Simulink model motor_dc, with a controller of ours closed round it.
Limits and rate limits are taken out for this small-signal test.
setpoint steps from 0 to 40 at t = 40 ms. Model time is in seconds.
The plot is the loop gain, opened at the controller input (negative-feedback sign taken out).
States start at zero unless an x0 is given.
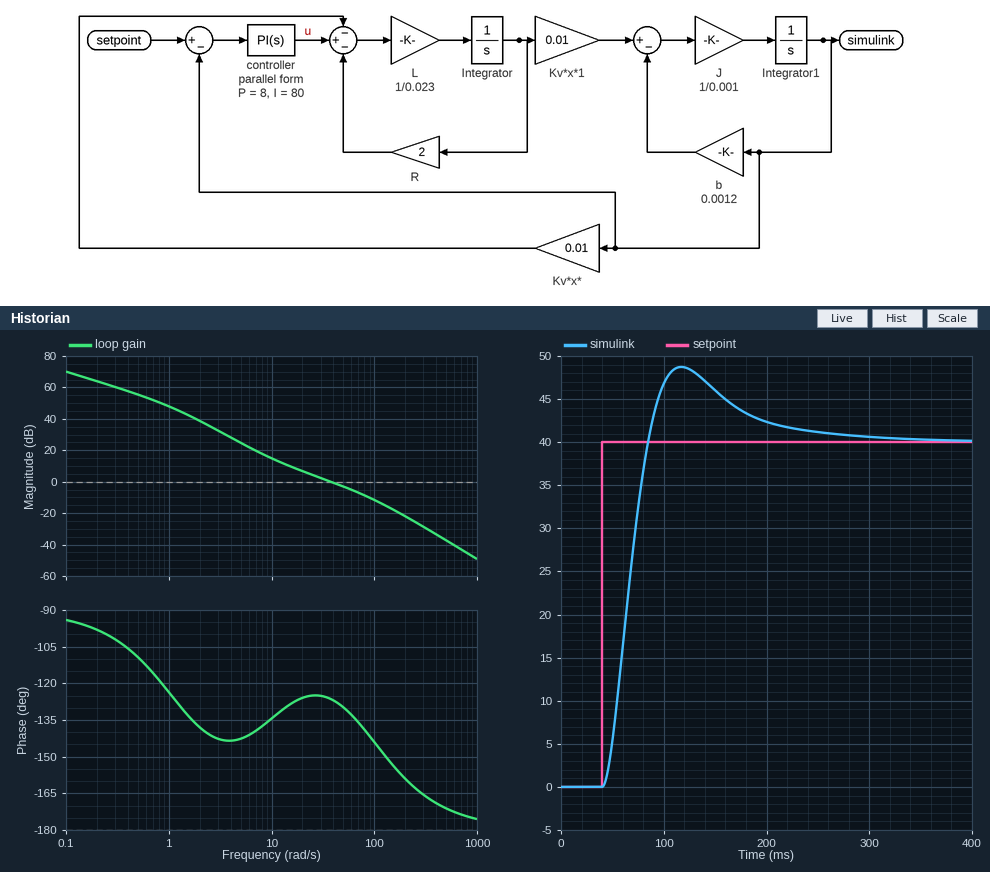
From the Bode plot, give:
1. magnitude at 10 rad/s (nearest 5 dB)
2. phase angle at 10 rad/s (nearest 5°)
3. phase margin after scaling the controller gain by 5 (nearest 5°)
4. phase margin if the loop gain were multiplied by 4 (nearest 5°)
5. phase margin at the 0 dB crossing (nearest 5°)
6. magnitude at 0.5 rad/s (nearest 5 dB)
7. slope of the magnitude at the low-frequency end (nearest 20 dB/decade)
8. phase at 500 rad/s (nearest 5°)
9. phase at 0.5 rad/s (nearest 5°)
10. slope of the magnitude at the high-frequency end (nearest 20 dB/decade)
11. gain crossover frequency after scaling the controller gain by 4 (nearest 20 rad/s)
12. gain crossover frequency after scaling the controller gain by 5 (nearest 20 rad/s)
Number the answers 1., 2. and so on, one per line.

1. 15 dB
2. -135°
3. 30°
4. 35°
5. 55°
6. 55 dB
7. -20 dB/decade
8. -170°
9. -110°
10. -40 dB/decade
11. 100 rad/s
12. 120 rad/s
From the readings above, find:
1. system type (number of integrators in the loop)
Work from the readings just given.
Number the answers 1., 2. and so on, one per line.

1. 1
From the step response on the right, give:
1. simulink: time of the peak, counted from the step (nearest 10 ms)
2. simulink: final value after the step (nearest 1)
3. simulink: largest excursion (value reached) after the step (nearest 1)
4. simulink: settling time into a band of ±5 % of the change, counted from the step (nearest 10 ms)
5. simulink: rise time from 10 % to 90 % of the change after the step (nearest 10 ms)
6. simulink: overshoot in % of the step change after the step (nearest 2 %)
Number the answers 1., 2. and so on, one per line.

1. 80 ms
2. 40
3. 49
4. 170 ms
5. 30 ms
6. 22 %
